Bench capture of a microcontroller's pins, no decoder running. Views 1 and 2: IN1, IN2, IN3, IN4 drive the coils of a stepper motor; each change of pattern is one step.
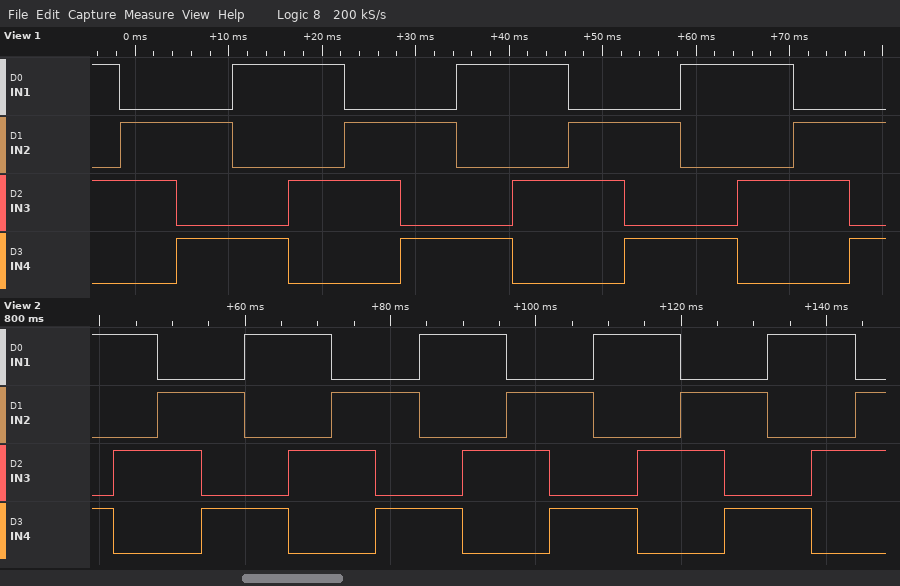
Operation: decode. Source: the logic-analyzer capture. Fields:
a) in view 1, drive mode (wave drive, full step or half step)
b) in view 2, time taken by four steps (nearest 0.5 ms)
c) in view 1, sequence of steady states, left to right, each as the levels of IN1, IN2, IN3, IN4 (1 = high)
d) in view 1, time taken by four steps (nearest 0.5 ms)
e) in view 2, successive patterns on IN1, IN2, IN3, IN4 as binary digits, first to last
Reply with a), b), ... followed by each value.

a) full step
b) 24.0 ms
c) 1010 0110 0101 1001 1010 0110 0101 1001 1010 0110 0101 1001 1010 0110 0101
d) 24.0 ms
e) 1001 1010 0110 0101 1001 1010 0110 0101 1001 1010 0110 0101 1001 1010 0110 0101 1001 1010 0110
